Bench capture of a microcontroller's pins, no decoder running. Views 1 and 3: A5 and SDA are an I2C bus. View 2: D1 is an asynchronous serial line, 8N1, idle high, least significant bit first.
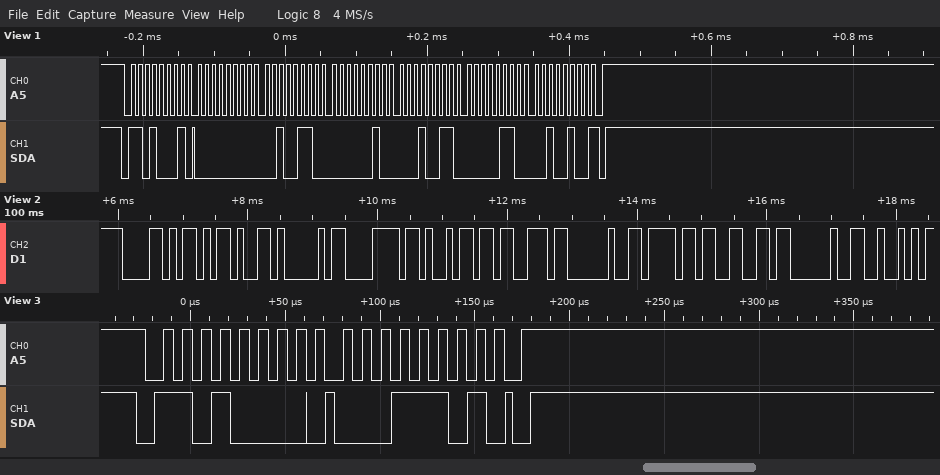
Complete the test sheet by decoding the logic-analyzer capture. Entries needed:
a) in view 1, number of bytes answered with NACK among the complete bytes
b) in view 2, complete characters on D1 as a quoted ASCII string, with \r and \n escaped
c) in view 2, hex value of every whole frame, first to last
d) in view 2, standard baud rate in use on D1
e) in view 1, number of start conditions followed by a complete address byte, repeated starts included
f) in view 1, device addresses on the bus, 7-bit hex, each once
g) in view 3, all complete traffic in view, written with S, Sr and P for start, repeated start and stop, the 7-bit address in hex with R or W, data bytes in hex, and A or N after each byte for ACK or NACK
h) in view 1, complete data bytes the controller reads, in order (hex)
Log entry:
1
"X-Axis of R"
58 2D 41 78 69 73 20 6F 66 20 52
9600 baud
1
0x68
S 68W A 1D A P
00 26 02 13 06 24
